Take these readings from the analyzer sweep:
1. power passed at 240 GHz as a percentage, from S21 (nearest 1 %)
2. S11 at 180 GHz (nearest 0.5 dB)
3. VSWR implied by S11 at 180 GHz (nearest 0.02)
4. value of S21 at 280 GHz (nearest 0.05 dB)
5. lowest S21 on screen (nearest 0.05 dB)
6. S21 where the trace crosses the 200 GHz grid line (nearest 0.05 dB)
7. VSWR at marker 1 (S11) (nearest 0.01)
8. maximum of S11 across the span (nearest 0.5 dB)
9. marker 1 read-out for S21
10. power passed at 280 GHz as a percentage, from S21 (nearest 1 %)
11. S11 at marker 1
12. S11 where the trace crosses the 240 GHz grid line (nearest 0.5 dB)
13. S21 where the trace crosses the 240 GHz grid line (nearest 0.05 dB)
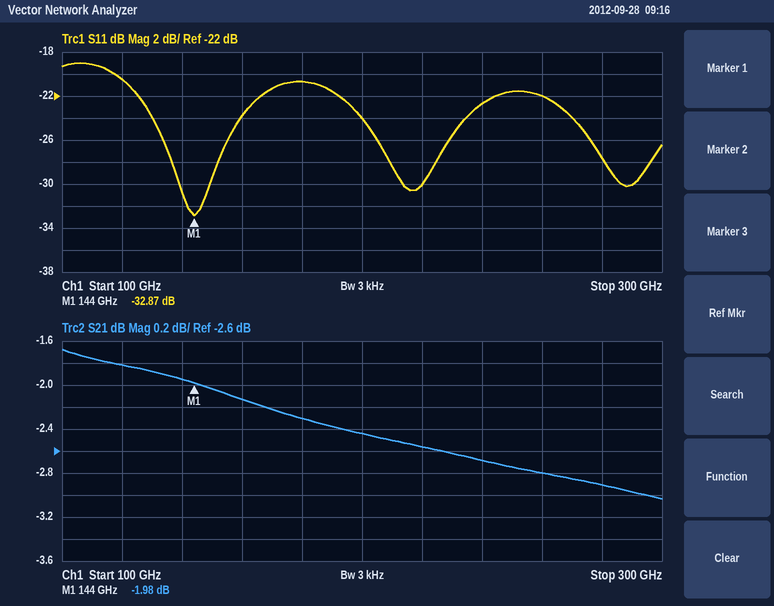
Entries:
54 %
-20.5 dB
1.20
-2.90 dB
-3.05 dB
-2.45 dB
1.05
-19.0 dB
-1.98 dB
51 %
-32.87 dB
-22.5 dB
-2.70 dB
